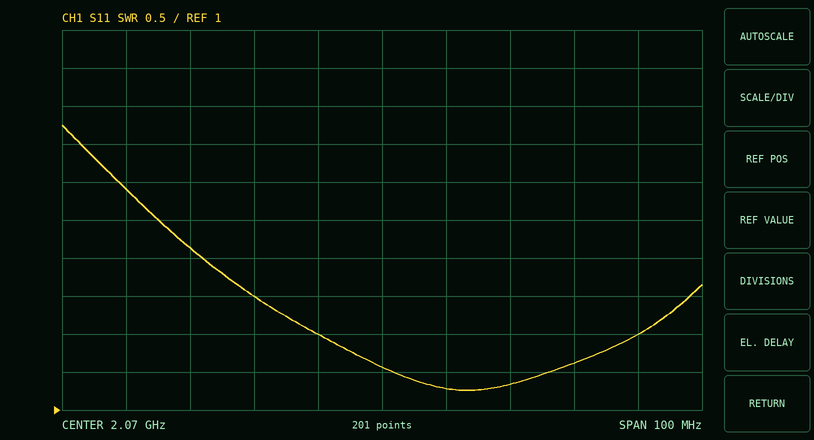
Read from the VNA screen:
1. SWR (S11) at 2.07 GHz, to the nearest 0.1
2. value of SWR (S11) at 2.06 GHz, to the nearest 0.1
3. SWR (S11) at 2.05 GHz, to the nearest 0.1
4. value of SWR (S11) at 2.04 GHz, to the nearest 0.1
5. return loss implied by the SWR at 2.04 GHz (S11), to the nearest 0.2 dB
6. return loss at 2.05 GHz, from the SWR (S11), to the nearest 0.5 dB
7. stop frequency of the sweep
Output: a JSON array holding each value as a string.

["1.6", "2.0", "2.5", "3.1", "5.8 dB", "7.5 dB", "2.12 GHz"]
